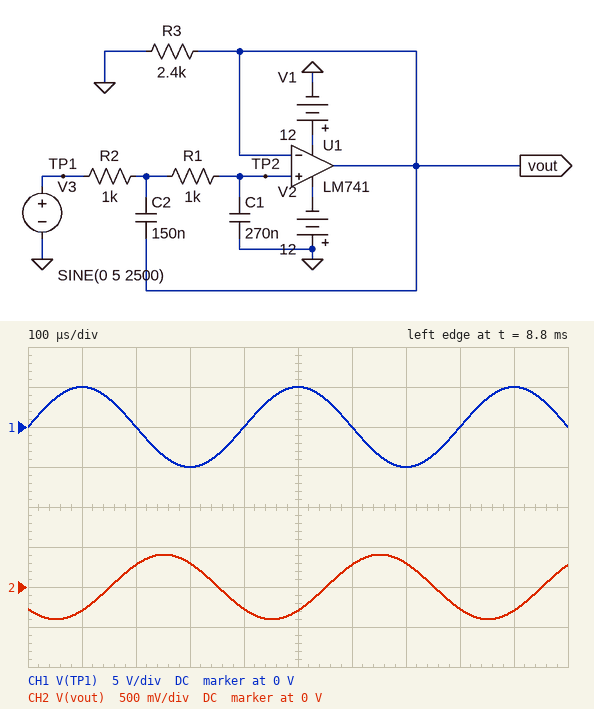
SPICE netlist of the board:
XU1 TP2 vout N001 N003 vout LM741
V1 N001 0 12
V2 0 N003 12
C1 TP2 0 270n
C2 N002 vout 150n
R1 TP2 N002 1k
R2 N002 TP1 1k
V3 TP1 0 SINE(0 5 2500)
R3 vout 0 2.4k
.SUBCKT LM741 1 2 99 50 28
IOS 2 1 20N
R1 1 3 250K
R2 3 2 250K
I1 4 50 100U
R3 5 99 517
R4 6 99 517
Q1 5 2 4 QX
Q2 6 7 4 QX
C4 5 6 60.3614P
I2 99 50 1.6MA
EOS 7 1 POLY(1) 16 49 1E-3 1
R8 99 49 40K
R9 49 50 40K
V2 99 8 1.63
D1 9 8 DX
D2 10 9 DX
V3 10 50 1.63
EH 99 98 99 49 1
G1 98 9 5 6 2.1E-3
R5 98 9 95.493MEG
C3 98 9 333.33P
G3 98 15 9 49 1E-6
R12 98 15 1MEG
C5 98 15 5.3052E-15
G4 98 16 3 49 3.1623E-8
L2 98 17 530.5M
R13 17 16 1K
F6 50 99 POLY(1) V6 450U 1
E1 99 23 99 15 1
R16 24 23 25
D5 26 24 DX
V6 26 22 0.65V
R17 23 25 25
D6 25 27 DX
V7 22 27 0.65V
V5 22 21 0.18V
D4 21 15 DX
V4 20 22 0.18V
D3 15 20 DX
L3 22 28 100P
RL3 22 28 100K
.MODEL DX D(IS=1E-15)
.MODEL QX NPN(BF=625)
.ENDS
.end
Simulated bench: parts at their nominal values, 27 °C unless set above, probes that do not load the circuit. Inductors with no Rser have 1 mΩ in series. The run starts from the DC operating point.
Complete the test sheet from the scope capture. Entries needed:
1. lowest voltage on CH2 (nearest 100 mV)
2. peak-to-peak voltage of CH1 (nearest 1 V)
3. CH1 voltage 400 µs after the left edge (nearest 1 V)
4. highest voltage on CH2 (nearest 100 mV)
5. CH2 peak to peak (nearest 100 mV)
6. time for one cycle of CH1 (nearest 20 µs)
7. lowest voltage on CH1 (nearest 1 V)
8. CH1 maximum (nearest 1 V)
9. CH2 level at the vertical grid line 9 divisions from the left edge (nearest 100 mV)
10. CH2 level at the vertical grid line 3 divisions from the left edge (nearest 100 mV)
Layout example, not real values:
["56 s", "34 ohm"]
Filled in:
["-400 mV", "10 V", "0 V", "400 mV", "800 mV", "400 µs", "-5 V", "5 V", "-300 mV", "300 mV"]
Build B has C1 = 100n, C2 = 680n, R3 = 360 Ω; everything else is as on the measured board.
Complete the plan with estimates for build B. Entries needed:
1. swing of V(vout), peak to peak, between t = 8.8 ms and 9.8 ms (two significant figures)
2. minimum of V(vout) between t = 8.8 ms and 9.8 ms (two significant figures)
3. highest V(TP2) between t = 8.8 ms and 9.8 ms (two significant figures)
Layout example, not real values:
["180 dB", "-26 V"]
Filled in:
["620 mV", "-310 mV", "310 mV"]
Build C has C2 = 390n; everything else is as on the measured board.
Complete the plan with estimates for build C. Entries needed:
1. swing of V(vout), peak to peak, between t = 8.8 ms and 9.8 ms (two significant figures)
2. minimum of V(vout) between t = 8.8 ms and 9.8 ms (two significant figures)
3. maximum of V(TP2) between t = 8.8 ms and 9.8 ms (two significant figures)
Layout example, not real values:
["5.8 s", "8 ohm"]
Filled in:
["380 mV", "-190 mV", "190 mV"]
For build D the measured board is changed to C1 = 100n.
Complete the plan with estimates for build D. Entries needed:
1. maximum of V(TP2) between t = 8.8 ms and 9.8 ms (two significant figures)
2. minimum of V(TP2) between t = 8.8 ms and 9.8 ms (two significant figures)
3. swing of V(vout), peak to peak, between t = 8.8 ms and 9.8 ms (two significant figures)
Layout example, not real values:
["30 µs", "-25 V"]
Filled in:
["1.2 V", "-1.2 V", "2.4 V"]
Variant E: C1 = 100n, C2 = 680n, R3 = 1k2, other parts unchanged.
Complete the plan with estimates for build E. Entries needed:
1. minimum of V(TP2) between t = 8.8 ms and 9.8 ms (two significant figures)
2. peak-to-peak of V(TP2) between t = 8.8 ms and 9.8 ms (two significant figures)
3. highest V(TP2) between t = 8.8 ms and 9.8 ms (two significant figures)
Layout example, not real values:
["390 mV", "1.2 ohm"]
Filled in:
["-310 mV", "620 mV", "310 mV"]
